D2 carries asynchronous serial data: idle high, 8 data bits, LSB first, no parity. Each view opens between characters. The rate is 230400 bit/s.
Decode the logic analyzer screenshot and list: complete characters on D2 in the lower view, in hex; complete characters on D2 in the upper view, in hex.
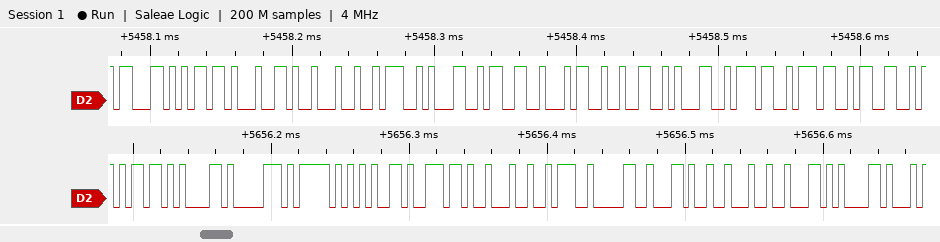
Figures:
6D, 61, 70, 5F, 65, 6E, 22, 3A, 30, 2C, 22, 62, 61
63, 6D, 64, 22, 3A, 31, 33, 34, 32, 31, 37, 37, 33
